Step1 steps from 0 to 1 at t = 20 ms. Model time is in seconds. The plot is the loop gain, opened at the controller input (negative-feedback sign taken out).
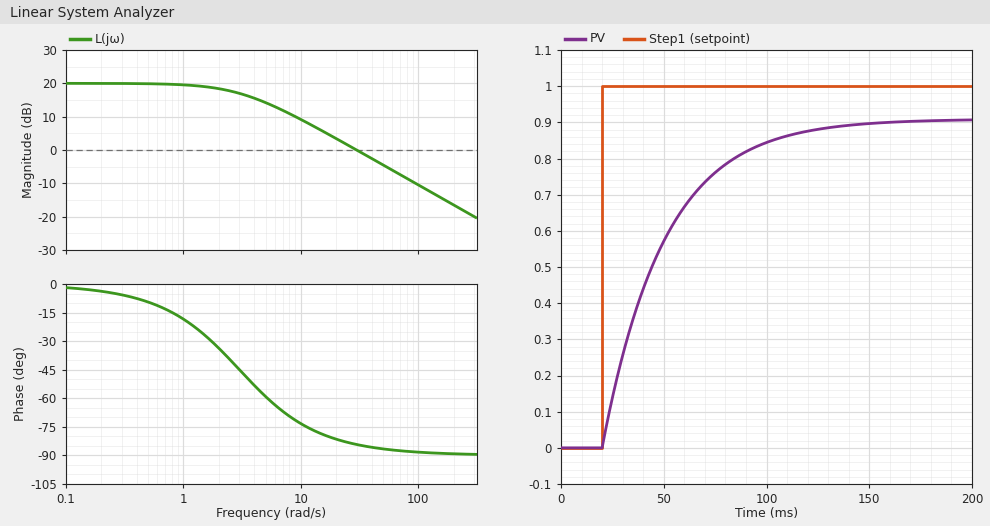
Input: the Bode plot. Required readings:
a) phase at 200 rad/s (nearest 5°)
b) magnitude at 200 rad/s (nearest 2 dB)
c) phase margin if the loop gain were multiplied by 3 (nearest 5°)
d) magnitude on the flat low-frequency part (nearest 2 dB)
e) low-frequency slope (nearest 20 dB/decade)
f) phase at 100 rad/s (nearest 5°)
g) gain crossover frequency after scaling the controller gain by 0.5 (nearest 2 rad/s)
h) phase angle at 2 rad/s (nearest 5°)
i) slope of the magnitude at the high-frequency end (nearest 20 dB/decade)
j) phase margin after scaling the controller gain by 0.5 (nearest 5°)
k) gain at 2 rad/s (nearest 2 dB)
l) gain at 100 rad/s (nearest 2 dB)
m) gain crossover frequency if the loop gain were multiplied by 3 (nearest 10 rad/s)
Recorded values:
-90°
-16 dB
90°
20 dB
0 dB/decade
-90°
14 rad/s
-35°
-20 dB/decade
100°
18 dB
-10 dB
90 rad/s
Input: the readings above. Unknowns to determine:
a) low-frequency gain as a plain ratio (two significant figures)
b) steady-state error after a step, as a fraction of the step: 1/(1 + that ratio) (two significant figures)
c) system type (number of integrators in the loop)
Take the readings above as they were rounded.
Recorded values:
10
0.091
0
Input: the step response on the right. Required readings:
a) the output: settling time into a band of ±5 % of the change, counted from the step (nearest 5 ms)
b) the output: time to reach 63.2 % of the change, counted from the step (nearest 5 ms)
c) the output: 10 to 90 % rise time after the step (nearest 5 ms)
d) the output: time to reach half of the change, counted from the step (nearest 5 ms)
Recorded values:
90 ms
30 ms
65 ms
20 ms
